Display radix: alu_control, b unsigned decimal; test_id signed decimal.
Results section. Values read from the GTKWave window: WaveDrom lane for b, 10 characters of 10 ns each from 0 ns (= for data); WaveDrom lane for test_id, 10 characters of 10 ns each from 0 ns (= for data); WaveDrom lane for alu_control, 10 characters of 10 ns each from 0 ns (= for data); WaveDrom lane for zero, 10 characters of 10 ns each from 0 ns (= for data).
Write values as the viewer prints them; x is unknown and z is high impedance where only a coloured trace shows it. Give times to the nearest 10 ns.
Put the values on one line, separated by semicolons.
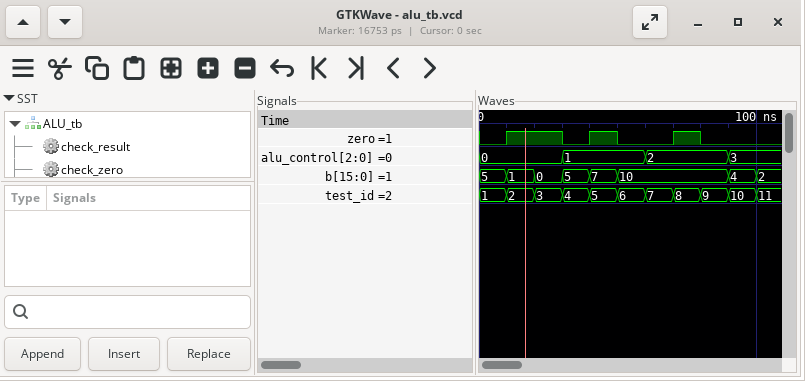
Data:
{name: 'b', wave: '======...=', data: '5 1 0 5 7 10 4'}; {name: 'test_id', wave: '==========', data: '1 2 3 4 5 6 7 8 9 10'}; {name: 'alu_control', wave: '=..=..=..=', data: '0 1 2 3'}; {name: 'zero', wave: '01.010.10.'}
